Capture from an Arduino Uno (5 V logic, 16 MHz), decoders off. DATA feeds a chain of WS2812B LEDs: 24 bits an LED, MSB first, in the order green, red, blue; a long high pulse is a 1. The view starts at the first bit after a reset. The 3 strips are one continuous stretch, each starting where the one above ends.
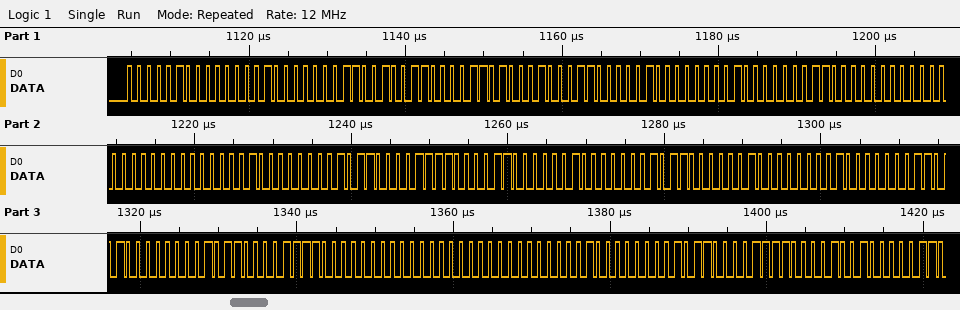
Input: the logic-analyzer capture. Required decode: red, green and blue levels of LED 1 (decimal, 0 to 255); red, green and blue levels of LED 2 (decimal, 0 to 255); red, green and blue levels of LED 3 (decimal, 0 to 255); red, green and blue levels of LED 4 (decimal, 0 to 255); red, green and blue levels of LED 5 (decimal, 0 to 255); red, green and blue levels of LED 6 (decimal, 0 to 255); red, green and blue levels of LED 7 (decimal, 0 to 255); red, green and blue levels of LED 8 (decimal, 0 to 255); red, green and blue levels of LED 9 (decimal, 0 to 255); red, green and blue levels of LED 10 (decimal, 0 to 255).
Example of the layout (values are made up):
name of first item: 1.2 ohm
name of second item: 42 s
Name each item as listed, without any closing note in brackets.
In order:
red, green and blue levels of LED 1: 2, 4, 3
red, green and blue levels of LED 2: 26, 38, 35
red, green and blue levels of LED 3: 2, 4, 3
red, green and blue levels of LED 4: 0, 0, 0
red, green and blue levels of LED 5: 22, 32, 30
red, green and blue levels of LED 6: 16, 24, 22
red, green and blue levels of LED 7: 2, 4, 3
red, green and blue levels of LED 8: 22, 32, 30
red, green and blue levels of LED 9: 0, 0, 0
red, green and blue levels of LED 10: 22, 32, 30
